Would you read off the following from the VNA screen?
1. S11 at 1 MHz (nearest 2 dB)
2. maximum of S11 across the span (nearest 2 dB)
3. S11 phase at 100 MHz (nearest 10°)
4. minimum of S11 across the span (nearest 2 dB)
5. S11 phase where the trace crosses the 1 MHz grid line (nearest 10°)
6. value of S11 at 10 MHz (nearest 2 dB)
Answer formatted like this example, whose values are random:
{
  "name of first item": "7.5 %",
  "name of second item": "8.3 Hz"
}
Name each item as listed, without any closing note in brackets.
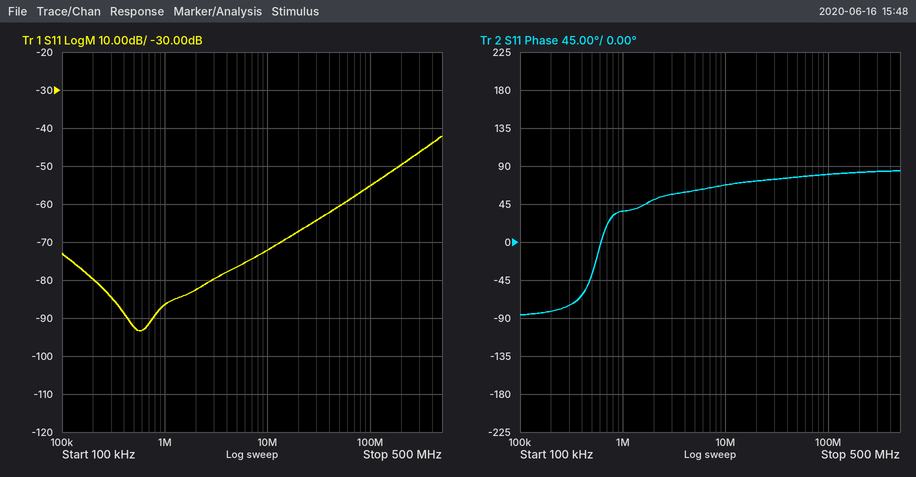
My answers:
{
  "S11 at 1 MHz": "-86 dB",
  "maximum of S11 across the span": "-42 dB",
  "S11 phase at 100 MHz": "80°",
  "minimum of S11 across the span": "-94 dB",
  "S11 phase where the trace crosses the 1 MHz grid line": "40°",
  "value of S11 at 10 MHz": "-72 dB"
}
